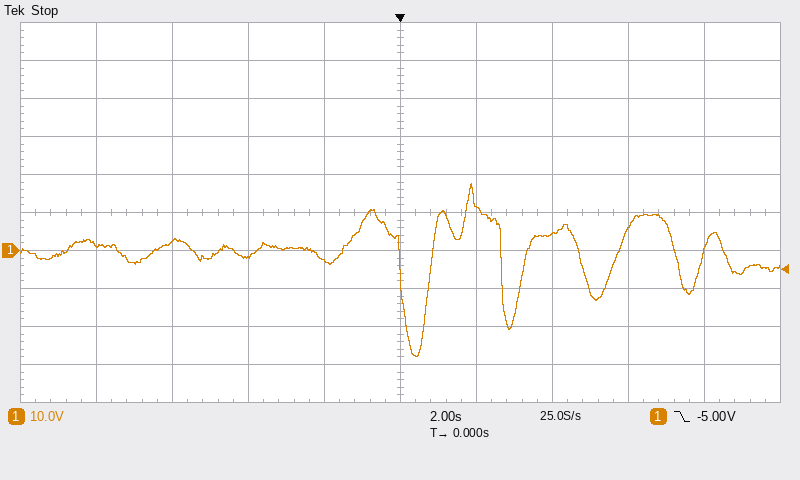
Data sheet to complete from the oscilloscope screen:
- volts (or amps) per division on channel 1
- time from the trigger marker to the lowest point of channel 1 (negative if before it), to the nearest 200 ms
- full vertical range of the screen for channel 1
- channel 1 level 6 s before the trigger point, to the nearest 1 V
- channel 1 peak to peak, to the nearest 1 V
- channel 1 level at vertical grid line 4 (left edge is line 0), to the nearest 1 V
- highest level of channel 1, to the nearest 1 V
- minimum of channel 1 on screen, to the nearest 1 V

10 V
+400 ms
100 V
2 V
46 V
-3 V
18 V
-28 V
